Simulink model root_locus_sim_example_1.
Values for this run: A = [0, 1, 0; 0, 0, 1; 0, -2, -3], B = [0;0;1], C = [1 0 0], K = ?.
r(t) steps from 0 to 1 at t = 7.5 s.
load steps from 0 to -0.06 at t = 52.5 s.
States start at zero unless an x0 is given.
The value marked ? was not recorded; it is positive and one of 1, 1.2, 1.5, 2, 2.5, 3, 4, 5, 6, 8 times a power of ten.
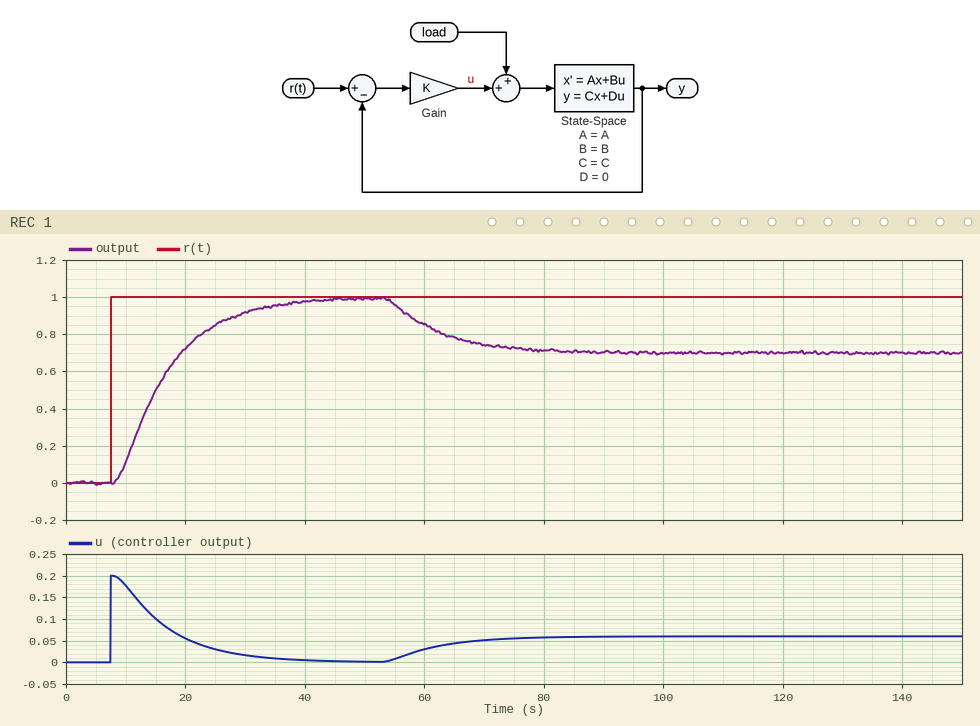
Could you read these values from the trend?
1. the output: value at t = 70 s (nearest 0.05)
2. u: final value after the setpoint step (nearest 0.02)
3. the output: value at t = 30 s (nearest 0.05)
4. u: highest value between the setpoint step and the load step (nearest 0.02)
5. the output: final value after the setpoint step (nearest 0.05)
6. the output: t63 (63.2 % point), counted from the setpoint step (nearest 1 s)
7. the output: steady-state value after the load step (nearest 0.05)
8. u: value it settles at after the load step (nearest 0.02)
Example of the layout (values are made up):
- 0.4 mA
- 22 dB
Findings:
- 0.75
- 0.00
- 0.90
- 0.20
- 1.00
- 10 s
- 0.70
- 0.06
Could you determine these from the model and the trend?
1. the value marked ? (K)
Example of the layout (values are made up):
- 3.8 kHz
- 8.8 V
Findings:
- 0.2
